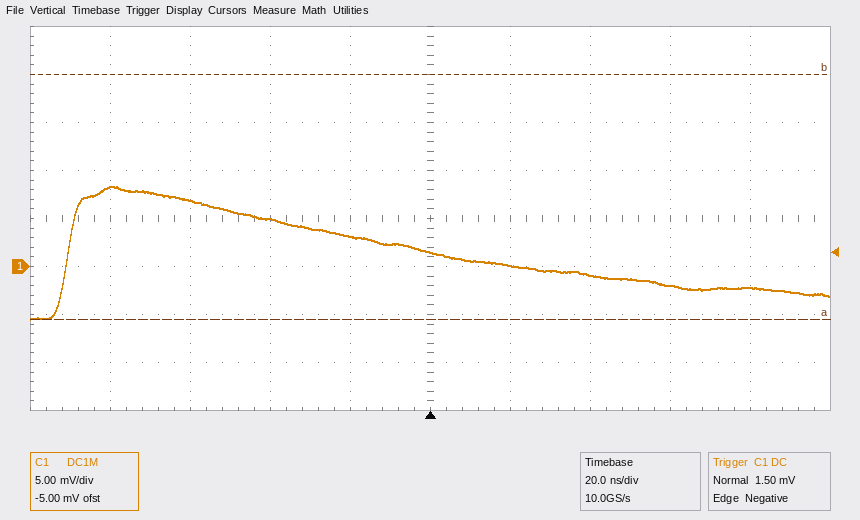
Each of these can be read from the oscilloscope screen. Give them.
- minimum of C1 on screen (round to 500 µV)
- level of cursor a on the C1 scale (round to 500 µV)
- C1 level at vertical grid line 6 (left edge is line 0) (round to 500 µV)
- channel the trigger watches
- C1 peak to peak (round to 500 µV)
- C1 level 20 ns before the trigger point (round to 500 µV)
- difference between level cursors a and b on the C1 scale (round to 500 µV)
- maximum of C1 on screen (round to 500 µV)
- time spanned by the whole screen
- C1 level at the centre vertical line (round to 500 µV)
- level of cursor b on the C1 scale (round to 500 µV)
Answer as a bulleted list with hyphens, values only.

- -5.5 mV
- -5.5 mV
- 0.0 mV
- C1
- 14.0 mV
- 3.0 mV
- 25.5 mV
- 8.5 mV
- 200 ns
- 1.5 mV
- 20.0 mV
